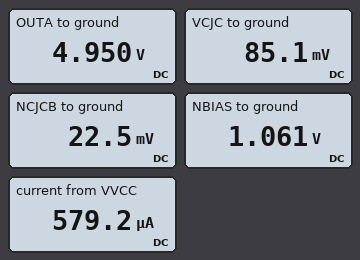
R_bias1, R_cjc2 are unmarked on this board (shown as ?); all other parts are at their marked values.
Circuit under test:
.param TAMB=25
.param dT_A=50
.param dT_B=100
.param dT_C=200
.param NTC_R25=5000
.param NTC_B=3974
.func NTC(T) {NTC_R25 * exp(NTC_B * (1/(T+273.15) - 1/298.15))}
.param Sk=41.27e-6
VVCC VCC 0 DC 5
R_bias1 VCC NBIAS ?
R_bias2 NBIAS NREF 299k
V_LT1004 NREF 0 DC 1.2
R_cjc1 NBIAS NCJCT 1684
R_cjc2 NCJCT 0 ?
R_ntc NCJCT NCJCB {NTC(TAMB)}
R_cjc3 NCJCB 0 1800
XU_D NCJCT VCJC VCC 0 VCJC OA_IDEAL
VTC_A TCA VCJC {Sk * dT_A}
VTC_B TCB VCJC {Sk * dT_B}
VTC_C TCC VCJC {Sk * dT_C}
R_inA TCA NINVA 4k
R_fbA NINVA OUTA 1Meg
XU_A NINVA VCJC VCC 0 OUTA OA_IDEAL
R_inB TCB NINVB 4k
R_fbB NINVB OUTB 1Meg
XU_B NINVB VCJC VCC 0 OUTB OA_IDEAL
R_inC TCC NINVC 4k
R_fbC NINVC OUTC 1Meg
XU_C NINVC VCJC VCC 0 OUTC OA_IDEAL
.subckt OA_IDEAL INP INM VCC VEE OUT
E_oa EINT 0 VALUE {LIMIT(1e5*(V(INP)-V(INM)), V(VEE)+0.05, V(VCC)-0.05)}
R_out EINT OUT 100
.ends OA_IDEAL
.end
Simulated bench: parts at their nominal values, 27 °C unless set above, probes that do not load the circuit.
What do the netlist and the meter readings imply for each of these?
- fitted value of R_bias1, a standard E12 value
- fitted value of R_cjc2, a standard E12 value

6.8 kΩ
150 Ω
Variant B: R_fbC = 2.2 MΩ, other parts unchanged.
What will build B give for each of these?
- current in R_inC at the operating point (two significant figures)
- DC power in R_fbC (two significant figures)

2.2 µA
11 µW
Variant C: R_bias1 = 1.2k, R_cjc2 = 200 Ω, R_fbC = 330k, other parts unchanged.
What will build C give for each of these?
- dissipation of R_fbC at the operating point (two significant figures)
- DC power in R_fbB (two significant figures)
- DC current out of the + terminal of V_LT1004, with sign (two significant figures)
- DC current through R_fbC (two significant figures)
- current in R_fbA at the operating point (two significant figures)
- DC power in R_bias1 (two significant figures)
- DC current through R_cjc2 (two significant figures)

63 µW
21 µW
-6.2 µA
14 µA
4.6 µA
3.2 mW
1.6 mA
